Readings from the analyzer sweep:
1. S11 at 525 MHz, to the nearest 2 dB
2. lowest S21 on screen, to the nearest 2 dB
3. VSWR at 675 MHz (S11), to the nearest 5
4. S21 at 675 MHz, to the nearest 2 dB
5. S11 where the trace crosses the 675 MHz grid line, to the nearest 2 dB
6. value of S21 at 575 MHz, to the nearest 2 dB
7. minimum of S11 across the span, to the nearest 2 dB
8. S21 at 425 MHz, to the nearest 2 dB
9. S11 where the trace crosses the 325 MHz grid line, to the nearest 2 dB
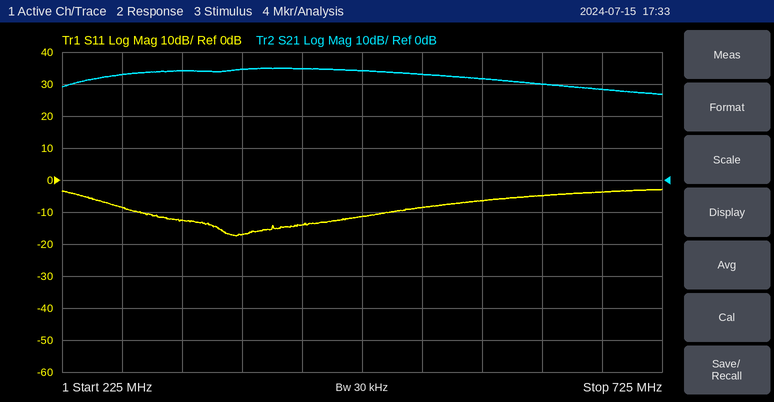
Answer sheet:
-8 dB
26 dB
5
28 dB
-4 dB
32 dB
-18 dB
34 dB
-12 dB
